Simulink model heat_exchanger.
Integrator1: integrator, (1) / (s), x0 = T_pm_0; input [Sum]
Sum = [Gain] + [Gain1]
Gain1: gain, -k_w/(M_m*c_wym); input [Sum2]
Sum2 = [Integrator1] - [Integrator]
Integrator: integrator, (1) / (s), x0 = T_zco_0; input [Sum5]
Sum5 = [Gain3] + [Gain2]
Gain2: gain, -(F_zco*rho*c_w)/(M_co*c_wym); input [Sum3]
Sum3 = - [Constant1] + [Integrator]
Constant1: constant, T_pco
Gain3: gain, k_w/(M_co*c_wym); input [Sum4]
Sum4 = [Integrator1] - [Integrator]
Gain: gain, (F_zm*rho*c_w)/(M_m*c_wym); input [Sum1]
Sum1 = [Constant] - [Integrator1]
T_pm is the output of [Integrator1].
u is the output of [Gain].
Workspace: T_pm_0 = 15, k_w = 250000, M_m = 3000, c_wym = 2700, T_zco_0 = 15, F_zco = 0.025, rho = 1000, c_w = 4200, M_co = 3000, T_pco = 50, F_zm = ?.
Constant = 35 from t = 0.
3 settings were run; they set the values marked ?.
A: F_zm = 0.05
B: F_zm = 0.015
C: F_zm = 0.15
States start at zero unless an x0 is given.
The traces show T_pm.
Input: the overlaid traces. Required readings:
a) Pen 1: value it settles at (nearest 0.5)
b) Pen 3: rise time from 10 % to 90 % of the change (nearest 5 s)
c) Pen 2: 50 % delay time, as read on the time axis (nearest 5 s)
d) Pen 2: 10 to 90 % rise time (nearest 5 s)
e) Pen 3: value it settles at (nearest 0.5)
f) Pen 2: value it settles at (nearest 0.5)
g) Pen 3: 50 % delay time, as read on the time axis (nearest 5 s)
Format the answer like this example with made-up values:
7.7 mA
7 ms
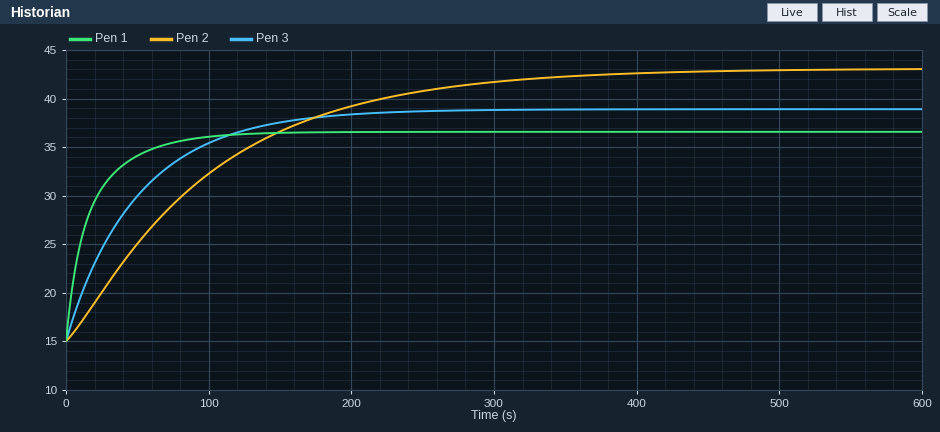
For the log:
36.5
115 s
75 s
215 s
39.0
43.0
35 s
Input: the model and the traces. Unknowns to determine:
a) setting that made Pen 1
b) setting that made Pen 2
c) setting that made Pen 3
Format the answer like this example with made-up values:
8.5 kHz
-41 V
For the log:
C
B
A
